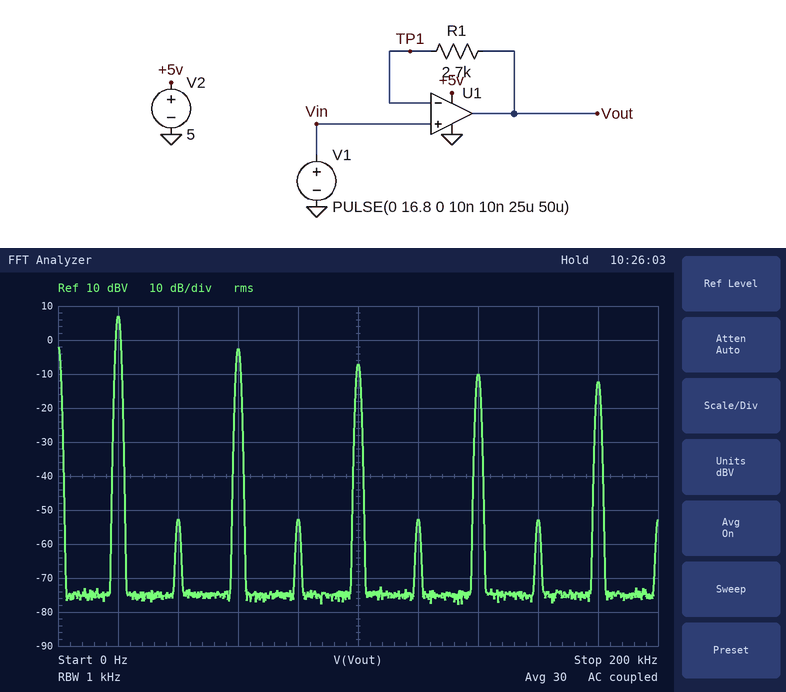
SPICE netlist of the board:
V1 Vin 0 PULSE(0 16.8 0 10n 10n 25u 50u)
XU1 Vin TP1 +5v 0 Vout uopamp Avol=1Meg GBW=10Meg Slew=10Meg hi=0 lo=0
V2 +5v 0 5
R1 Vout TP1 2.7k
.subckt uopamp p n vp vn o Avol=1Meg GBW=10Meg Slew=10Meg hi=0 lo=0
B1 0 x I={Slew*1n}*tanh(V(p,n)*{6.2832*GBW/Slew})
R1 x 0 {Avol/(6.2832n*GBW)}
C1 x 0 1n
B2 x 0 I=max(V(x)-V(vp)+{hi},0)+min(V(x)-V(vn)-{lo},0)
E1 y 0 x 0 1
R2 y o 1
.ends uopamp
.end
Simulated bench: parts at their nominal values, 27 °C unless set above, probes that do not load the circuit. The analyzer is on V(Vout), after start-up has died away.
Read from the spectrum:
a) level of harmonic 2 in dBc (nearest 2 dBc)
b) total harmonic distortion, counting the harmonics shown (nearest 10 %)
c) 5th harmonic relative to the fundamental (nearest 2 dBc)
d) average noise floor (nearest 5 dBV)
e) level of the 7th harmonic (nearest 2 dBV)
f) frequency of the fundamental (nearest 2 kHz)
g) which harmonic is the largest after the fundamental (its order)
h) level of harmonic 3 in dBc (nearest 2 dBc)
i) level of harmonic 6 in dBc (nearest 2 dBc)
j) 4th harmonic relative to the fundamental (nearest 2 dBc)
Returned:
-60 dBc
40 %
-14 dBc
-75 dBV
-10 dBV
20 kHz
3
-10 dBc
-60 dBc
-60 dBc
